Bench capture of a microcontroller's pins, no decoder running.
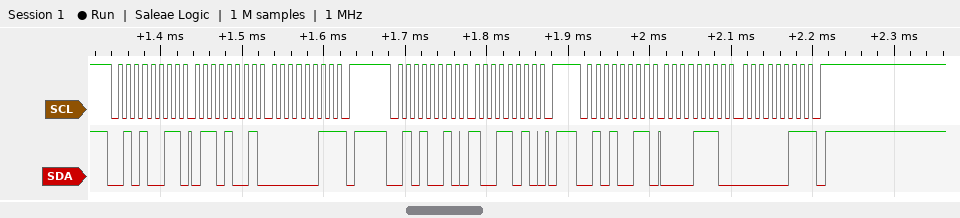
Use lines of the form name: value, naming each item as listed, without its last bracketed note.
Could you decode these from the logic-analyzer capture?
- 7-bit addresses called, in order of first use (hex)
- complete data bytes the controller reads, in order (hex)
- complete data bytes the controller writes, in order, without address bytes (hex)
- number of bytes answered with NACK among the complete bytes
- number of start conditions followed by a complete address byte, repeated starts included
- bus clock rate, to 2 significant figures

7-bit addresses called, in order of first use: 0x29
complete data bytes the controller reads, in order: 69 03 0E 03
complete data bytes the controller writes, in order, without address bytes: 9A
number of bytes answered with NACK among the complete bytes: 2
number of start conditions followed by a complete address byte, repeated starts included: 3
bus clock rate, to 2 significant figures: 100 kHz
